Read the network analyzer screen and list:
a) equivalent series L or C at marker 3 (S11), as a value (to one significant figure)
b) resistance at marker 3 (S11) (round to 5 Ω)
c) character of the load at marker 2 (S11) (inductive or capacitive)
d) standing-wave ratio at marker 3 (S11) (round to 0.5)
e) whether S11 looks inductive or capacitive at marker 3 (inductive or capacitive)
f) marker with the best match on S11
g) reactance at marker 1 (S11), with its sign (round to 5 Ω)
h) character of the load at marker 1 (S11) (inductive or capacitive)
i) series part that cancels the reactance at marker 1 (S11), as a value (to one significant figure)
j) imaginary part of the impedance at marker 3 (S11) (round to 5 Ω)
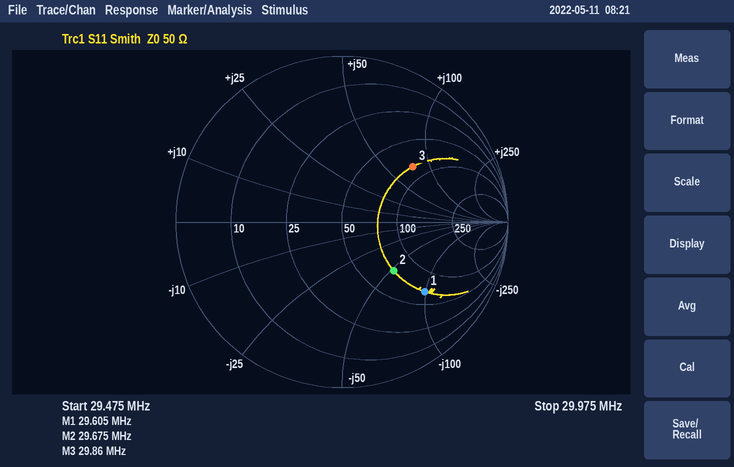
400 nH
80 Ω
capacitive
3.5
inductive
marker 2
-100 Ω
capacitive
500 nH
+75 Ω
